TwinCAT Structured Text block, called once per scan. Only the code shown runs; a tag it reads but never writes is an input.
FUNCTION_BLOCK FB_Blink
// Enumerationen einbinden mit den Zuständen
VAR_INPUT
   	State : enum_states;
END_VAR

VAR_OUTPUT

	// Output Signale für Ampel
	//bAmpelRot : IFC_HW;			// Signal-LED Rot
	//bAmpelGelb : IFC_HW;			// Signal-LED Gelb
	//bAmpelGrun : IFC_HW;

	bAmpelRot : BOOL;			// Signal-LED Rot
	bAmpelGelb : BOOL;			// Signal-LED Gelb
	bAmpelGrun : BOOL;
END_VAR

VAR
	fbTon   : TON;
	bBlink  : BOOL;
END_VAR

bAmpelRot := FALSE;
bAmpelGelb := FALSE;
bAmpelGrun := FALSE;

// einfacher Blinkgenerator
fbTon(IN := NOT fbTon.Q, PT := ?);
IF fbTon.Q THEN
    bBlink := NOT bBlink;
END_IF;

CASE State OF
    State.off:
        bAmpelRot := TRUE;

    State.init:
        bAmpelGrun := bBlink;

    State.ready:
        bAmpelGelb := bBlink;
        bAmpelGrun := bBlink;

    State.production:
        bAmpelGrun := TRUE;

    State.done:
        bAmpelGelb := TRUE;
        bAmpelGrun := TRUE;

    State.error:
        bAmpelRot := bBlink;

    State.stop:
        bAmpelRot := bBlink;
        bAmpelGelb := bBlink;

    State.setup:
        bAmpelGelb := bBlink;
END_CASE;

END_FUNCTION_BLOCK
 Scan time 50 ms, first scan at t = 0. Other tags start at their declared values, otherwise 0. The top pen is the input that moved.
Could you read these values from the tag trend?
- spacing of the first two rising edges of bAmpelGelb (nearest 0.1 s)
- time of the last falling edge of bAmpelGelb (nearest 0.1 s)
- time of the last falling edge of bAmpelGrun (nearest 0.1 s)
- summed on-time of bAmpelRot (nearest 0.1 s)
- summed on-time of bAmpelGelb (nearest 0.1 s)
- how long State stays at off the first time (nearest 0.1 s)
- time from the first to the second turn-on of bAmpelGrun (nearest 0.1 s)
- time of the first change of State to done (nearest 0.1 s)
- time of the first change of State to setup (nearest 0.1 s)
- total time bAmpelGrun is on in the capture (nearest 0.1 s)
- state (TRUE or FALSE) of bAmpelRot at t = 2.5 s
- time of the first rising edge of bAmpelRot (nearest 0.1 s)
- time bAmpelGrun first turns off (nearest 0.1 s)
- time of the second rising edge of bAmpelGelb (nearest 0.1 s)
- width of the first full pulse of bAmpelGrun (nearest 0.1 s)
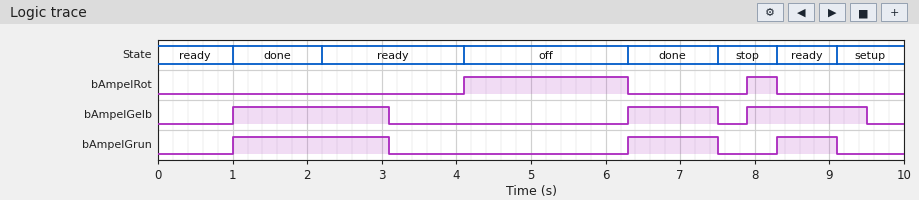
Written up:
5.3 s
9.5 s
9.1 s
2.6 s
4.9 s
2.2 s
5.3 s
1.0 s
9.1 s
4.1 s
FALSE
4.1 s
3.1 s
6.3 s
2.1 s
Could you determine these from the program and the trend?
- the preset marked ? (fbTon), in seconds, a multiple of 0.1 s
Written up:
1.5 s
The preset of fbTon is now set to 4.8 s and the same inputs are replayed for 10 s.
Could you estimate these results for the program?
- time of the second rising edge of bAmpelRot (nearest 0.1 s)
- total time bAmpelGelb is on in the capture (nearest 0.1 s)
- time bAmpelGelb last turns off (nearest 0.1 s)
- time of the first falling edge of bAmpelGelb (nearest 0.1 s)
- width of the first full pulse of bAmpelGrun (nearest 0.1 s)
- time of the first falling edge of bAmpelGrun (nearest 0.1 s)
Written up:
7.5 s
4.6 s
9.7 s
2.2 s
1.2 s
2.2 s
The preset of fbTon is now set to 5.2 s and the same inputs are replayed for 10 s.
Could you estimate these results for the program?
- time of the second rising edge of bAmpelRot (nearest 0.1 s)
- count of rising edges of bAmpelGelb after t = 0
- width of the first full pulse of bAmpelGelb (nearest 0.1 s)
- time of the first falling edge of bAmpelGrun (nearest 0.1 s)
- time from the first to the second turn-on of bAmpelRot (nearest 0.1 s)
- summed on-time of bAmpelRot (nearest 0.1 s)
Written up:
7.5 s
2
1.2 s
2.2 s
3.4 s
3.0 s
